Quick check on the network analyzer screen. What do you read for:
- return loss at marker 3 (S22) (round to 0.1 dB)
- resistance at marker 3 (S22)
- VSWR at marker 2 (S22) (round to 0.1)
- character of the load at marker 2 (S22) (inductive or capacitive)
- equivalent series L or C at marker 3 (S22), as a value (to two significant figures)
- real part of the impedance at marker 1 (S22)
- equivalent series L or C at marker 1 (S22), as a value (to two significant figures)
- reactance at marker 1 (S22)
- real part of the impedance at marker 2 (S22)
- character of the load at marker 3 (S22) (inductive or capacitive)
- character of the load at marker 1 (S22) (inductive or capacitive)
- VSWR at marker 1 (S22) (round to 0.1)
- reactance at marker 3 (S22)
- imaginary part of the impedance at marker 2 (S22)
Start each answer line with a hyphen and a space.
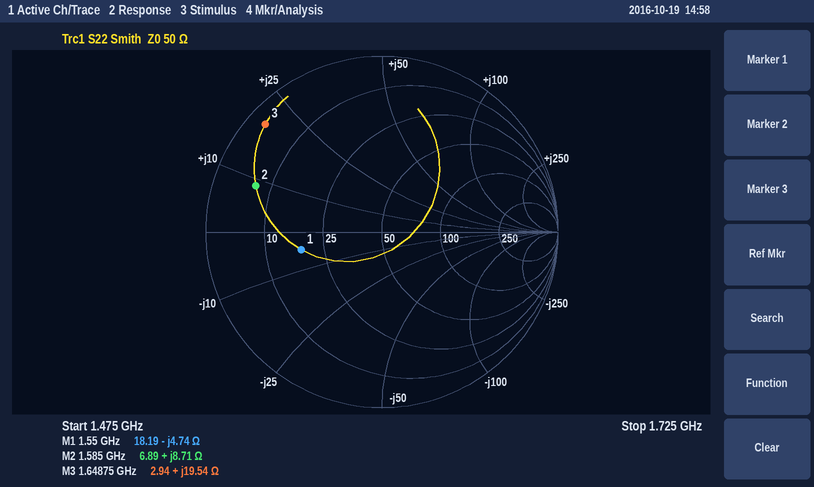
- 0.9 dB
- 2.94 Ω
- 7.5
- inductive
- 1.9 nH
- 18.19 Ω
- 22 pF
- -4.74 Ω
- 6.89 Ω
- inductive
- capacitive
- 2.8
- +19.54 Ω
- +8.71 Ω
